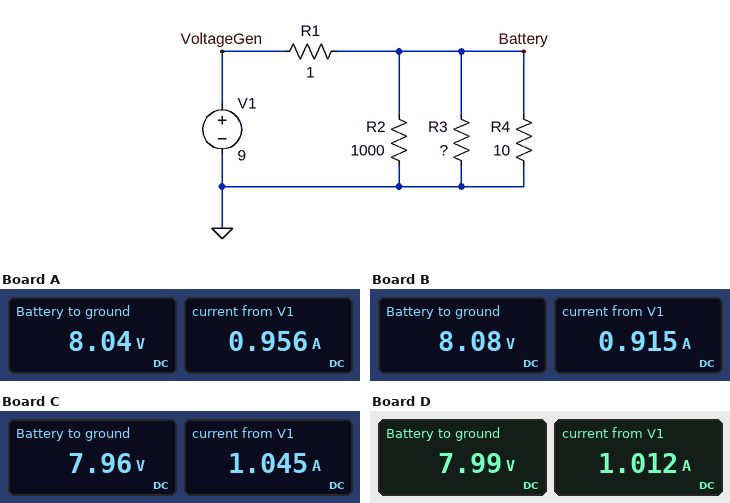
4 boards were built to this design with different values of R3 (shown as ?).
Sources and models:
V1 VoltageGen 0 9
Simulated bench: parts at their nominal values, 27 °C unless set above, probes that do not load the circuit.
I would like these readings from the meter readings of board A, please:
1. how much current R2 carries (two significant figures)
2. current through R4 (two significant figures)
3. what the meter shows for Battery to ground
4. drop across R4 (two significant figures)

8.0 mA
800 mA
8.04 V
8.0 V
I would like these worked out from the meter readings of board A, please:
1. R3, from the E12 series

56 Ω
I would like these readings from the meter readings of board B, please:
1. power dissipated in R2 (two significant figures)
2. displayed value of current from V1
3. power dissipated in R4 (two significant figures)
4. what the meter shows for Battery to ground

65 mW
0.915 A
6.5 W
8.08 V
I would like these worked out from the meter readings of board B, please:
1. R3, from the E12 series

82 Ω
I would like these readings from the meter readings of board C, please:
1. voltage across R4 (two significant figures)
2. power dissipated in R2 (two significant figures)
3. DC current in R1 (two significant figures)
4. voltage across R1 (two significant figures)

8.0 V
63 mW
1.0 A
1.0 V
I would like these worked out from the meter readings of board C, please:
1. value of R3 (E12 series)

33 Ω
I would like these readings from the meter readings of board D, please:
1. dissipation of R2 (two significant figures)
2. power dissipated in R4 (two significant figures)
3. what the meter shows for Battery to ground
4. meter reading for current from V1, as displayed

64 mW
6.4 W
7.99 V
1.012 A
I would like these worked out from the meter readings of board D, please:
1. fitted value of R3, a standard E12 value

39 Ω
